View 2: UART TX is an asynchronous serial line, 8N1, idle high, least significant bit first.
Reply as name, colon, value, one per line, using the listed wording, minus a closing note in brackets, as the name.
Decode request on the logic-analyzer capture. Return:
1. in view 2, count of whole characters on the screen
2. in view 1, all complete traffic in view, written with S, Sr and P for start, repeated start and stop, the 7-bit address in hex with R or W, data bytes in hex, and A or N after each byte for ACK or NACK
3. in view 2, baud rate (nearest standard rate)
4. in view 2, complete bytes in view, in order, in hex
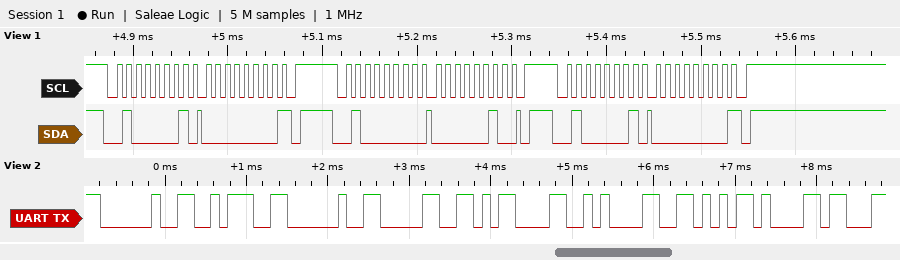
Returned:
in view 2, count of whole characters on the screen: 8
in view 1, all complete traffic in view, written with S, Sr and P for start, repeated start and stop, the 7-bit address in hex with R or W, data bytes in hex, and A or N after each byte for ACK or NACK: S 20R A 00 N P S 20W A 02 A P S 20R A 00 N P
in view 2, baud rate: 9600 baud
in view 2, complete bytes in view, in order, in hex: 20 3A 20 30 0D 0A 56 61
